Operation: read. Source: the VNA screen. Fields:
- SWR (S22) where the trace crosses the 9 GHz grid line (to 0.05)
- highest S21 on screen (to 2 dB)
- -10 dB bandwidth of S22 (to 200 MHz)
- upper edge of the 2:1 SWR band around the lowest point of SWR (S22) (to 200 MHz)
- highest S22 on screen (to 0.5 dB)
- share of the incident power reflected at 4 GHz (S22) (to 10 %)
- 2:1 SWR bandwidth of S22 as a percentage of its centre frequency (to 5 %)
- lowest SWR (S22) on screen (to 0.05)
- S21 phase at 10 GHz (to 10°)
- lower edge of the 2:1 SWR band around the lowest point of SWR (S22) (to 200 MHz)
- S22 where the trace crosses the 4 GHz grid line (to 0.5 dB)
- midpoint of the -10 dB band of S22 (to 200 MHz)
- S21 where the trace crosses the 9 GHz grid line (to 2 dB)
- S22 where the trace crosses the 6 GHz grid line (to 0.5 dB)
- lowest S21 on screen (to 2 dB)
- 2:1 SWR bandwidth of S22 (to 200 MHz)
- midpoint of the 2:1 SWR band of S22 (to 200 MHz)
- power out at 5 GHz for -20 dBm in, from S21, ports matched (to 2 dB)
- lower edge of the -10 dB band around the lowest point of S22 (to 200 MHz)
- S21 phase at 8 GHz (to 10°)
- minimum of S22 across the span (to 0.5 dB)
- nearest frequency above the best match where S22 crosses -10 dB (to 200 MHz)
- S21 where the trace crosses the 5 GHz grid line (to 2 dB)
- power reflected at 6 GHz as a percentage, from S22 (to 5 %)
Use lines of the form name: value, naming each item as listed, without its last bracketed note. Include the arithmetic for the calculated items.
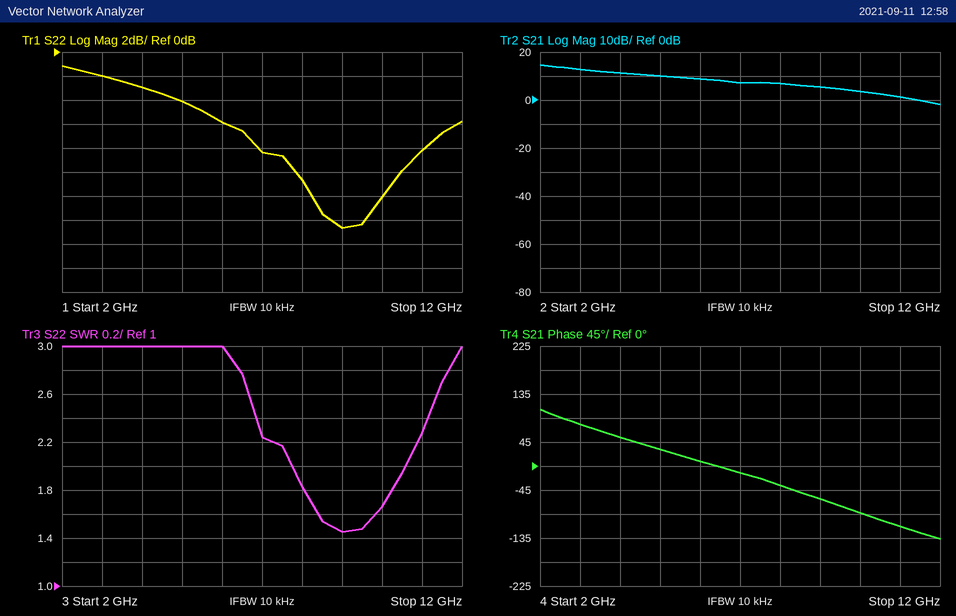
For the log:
SWR (S22) where the trace crosses the 9 GHz grid line: 1.45
highest S21 on screen: 14 dB
-10 dB bandwidth of S22: 10.4 GHz − 7.8 GHz = 2.6 GHz
upper edge of the 2:1 SWR band around the lowest point of SWR (S22): 10.6 GHz
highest S22 on screen: -1.0 dB
share of the incident power reflected at 4 GHz (S22): 10^(-3/10) ≈ 50 %
2:1 SWR bandwidth of S22 as a percentage of its centre frequency: 2.8 GHz / 9.2 GHz ≈ 30 %
lowest SWR (S22) on screen: 1.45
S21 phase at 10 GHz: -90°
lower edge of the 2:1 SWR band around the lowest point of SWR (S22): 7.8 GHz
S22 where the trace crosses the 4 GHz grid line: -3.0 dB
midpoint of the -10 dB band of S22: 9.2 GHz
S21 where the trace crosses the 9 GHz grid line: 6 dB
S22 where the trace crosses the 6 GHz grid line: -6.0 dB
lowest S21 on screen: -2 dB
2:1 SWR bandwidth of S22: 10.6 GHz − 7.8 GHz = 2.8 GHz
midpoint of the 2:1 SWR band of S22: 9.2 GHz
power out at 5 GHz for -20 dBm in, from S21, ports matched: -20 dBm + (10 dB) = -10 dBm
lower edge of the -10 dB band around the lowest point of S22: 7.8 GHz
S21 phase at 8 GHz: -40°
minimum of S22 across the span: -14.5 dB
nearest frequency above the best match where S22 crosses -10 dB: 10.4 GHz
S21 where the trace crosses the 5 GHz grid line: 10 dB
power reflected at 6 GHz as a percentage, from S22: 10^(-6/10) ≈ 25 %
